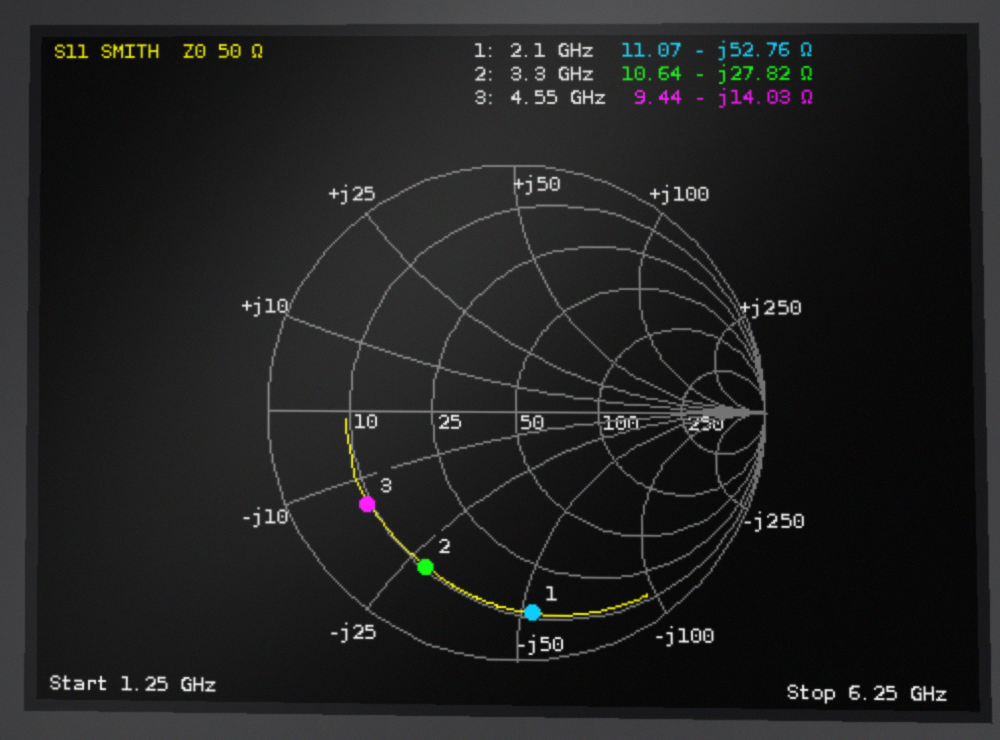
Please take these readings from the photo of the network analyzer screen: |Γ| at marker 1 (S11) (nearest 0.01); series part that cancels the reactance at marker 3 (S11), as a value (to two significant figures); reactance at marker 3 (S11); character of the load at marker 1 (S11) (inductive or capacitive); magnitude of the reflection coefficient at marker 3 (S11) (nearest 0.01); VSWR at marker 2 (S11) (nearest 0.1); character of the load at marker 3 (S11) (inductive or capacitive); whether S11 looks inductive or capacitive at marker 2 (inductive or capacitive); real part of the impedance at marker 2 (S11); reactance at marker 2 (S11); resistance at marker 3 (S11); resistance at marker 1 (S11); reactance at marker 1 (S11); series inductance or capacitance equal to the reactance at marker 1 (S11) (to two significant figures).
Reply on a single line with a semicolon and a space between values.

0.81; 490 pH; -14.03 Ω; capacitive; 0.70; 6.2; capacitive; capacitive; 10.64 Ω; -27.82 Ω; 9.44 Ω; 11.07 Ω; -52.76 Ω; 1.4 pF
